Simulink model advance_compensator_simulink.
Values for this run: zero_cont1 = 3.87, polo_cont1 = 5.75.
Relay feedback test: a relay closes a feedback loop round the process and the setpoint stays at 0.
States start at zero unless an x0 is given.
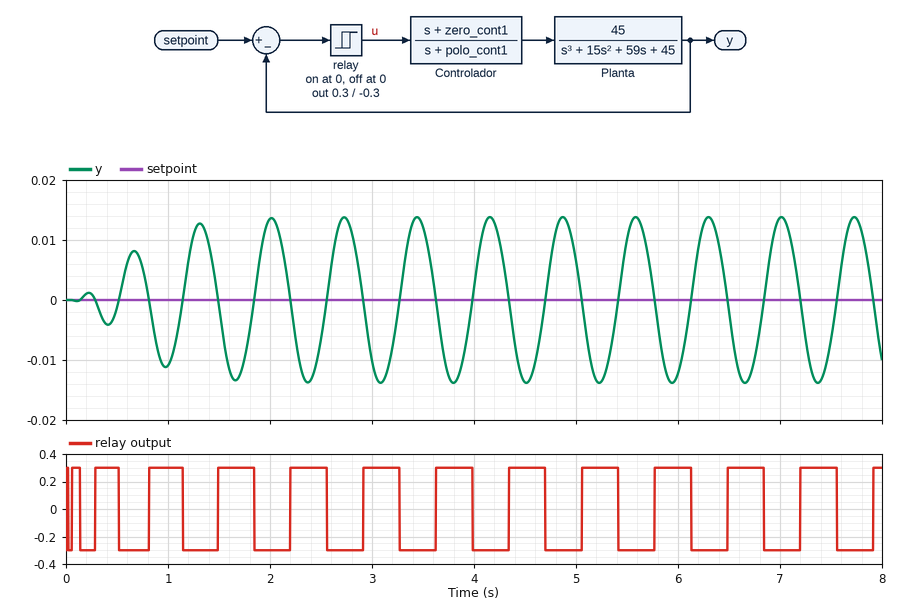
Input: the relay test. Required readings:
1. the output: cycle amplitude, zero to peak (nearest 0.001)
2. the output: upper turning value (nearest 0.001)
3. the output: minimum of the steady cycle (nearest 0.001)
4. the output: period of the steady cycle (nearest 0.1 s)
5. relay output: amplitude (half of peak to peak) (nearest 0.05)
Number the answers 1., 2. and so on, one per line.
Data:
1. 0.014
2. 0.014
3. -0.014
4. 0.7 s
5. 0.30
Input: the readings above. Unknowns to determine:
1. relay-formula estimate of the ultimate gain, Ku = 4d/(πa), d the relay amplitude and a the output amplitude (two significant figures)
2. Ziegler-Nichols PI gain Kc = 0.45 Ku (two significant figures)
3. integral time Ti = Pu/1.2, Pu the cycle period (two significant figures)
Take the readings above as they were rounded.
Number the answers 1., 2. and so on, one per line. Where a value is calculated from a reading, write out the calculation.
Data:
1. 4 × 0.3 / (π × 0.014) = 27
2. 0.45 × 27 = 12
3. 0.7 / 1.2 = 0.58 s
